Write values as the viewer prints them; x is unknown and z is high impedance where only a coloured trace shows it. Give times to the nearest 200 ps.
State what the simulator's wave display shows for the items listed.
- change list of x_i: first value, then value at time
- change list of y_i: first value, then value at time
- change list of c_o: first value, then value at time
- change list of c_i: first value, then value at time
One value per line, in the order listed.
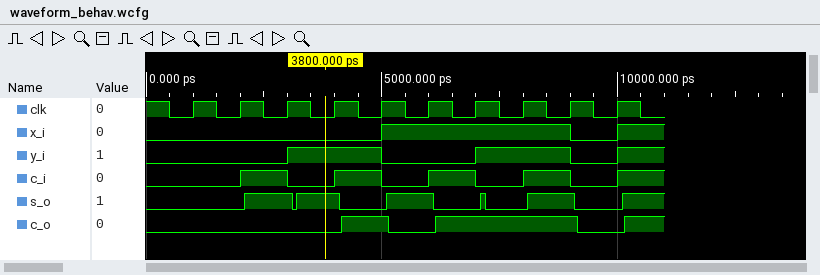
0, 1 at 5000 ps, 0 at 9000 ps, 1 at 10000 ps
0, 1 at 3000 ps, 0 at 5000 ps, 1 at 7000 ps, 0 at 9000 ps, 1 at 10000 ps
0, 1 at 4200 ps, 0 at 5200 ps, 1 at 6200 ps, 0 at 9200 ps, 1 at 10200 ps
0, 1 at 2000 ps, 0 at 3000 ps, 1 at 4000 ps, 0 at 5000 ps, 1 at 6000 ps, 0 at 7000 ps, 1 at 8000 ps, 0 at 9000 ps, 1 at 10000 ps
